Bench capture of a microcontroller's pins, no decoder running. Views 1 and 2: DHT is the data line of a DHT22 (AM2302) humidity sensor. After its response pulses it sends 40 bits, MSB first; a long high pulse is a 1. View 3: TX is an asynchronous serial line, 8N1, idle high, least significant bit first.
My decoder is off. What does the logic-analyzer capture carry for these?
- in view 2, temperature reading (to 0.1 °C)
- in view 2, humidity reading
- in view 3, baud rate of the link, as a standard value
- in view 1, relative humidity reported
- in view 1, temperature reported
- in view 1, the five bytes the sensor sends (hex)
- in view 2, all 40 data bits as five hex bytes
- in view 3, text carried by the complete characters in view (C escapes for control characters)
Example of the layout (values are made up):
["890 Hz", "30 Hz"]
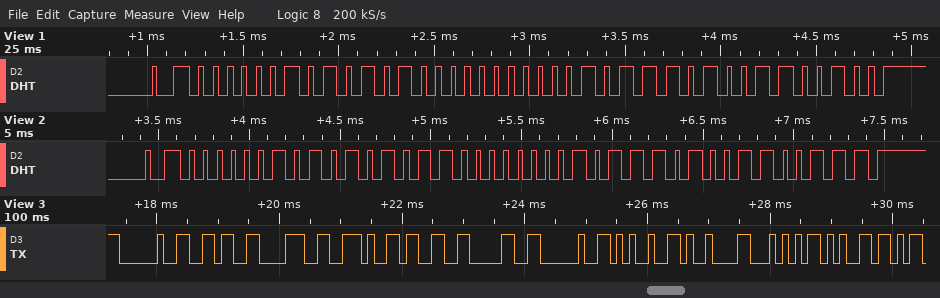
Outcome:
["18.6 °C", "68.3 %", "9600 baud", "68.0 %", "18.6 °C", "02 A8 00 BA 64", "02 AB 00 BA 67", "\" 68.30 %\\tTe\""]
